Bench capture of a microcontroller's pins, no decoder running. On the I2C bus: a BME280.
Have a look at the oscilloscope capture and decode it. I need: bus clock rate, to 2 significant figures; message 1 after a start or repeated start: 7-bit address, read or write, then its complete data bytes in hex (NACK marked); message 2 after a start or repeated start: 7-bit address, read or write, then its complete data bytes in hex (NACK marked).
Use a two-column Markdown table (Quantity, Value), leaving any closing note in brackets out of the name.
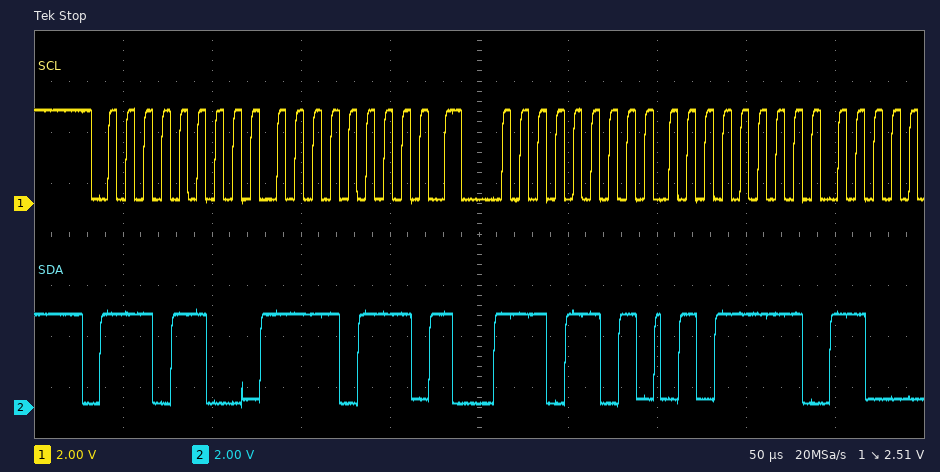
| Quantity | Value |
|---|---|
| bus clock rate, to 2 significant figures | 100 kHz |
| message 1 after a start or repeated start: 7-bit address, read or write, then its complete data bytes in hex | 0x76 write: F7 |
| message 2 after a start or repeated start: 7-bit address, read or write, then its complete data bytes in hex | 0x76 read: 5F |
